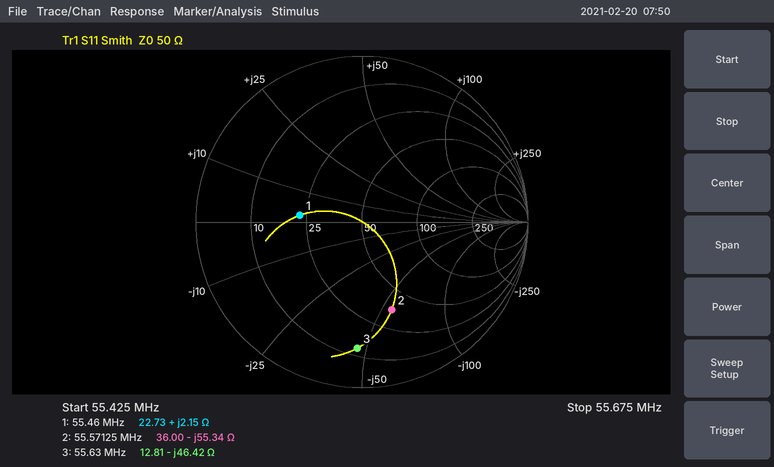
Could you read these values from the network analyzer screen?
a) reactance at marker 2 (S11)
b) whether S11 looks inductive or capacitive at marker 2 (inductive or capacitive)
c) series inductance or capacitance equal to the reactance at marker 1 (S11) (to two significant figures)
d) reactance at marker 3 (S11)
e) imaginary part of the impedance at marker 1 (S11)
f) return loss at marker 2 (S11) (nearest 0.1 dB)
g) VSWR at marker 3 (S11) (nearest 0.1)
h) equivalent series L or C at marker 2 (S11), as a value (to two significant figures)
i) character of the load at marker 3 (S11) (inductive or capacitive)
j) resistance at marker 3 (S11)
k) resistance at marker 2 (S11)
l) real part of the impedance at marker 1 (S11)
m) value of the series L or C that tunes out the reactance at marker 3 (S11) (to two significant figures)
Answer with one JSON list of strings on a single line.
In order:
["-55.34 Ω", "capacitive", "6.2 nH", "-46.42 Ω", "+2.15 Ω", "5.1 dB", "7.4", "52 pF", "capacitive", "12.81 Ω", "36.00 Ω", "22.73 Ω", "130 nH"]
